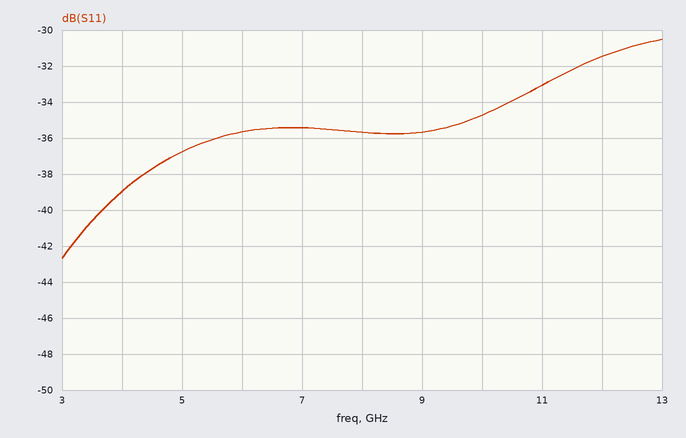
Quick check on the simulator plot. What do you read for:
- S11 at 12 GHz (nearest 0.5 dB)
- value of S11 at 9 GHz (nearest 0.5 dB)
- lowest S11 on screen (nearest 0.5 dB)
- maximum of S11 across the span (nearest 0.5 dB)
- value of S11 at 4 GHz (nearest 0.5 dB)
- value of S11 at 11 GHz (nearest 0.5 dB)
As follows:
-31.5 dB
-35.5 dB
-42.5 dB
-30.5 dB
-39.0 dB
-33.0 dB
